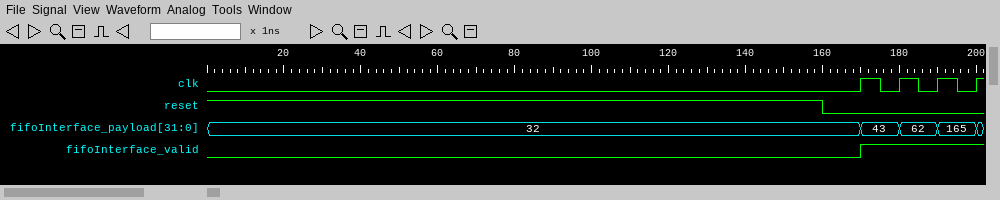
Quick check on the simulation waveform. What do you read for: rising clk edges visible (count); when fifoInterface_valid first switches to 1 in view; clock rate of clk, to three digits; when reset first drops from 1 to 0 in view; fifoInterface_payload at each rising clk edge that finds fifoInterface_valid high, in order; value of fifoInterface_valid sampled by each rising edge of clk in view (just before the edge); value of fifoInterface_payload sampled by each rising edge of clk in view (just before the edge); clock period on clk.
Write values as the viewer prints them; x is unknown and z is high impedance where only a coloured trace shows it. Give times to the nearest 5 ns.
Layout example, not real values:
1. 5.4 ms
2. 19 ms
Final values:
1. 4
2. 170 ns
3. 100 MHz
4. 160 ns
5. 43, 62, 165
6. 0 1 1 1
7. 32, 43, 62, 165
8. 10 ns
